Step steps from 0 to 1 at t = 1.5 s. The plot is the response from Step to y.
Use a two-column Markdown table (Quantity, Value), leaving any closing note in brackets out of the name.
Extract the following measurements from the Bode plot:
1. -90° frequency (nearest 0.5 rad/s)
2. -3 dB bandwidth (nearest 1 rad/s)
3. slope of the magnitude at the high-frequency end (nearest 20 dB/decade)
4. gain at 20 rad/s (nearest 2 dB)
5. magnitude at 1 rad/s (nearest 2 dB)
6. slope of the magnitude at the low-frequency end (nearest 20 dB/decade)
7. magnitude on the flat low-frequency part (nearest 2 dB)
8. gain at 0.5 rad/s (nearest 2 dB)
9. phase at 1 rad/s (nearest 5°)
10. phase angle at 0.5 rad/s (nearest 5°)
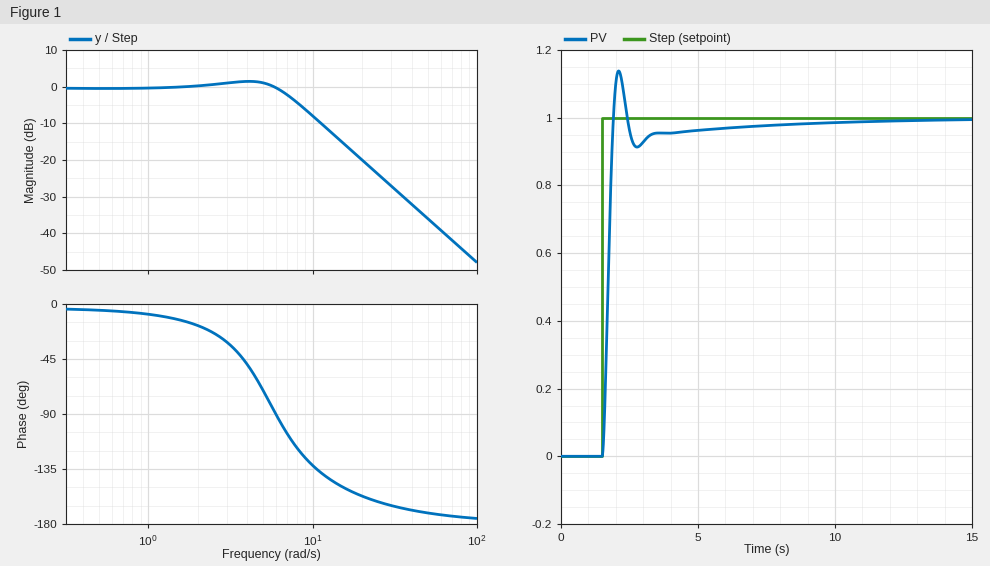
| Quantity | Value |
|---|---|
| -90° frequency | 6.0 rad/s |
| -3 dB bandwidth | 8 rad/s |
| slope of the magnitude at the high-frequency end | -40 dB/decade |
| gain at 20 rad/s | -20 dB |
| magnitude at 1 rad/s | 0 dB |
| slope of the magnitude at the low-frequency end | 0 dB/decade |
| magnitude on the flat low-frequency part | 0 dB |
| gain at 0.5 rad/s | 0 dB |
| phase at 1 rad/s | -10° |
| phase angle at 0.5 rad/s | -5° |
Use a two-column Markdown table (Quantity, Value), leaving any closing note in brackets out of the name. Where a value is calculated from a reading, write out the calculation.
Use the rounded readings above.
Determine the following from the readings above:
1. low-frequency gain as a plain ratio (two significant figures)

| Quantity | Value |
|---|---|
| low-frequency gain as a plain ratio | 10^(0 / 20) = 1.0 |
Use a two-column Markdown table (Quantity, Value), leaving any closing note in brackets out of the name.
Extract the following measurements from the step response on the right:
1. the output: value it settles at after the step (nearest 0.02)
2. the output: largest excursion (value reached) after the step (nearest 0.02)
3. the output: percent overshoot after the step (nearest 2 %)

| Quantity | Value |
|---|---|
| the output: value it settles at after the step | 1.00 |
| the output: largest excursion (value reached) after the step | 1.14 |
| the output: percent overshoot after the step | 14 % |
